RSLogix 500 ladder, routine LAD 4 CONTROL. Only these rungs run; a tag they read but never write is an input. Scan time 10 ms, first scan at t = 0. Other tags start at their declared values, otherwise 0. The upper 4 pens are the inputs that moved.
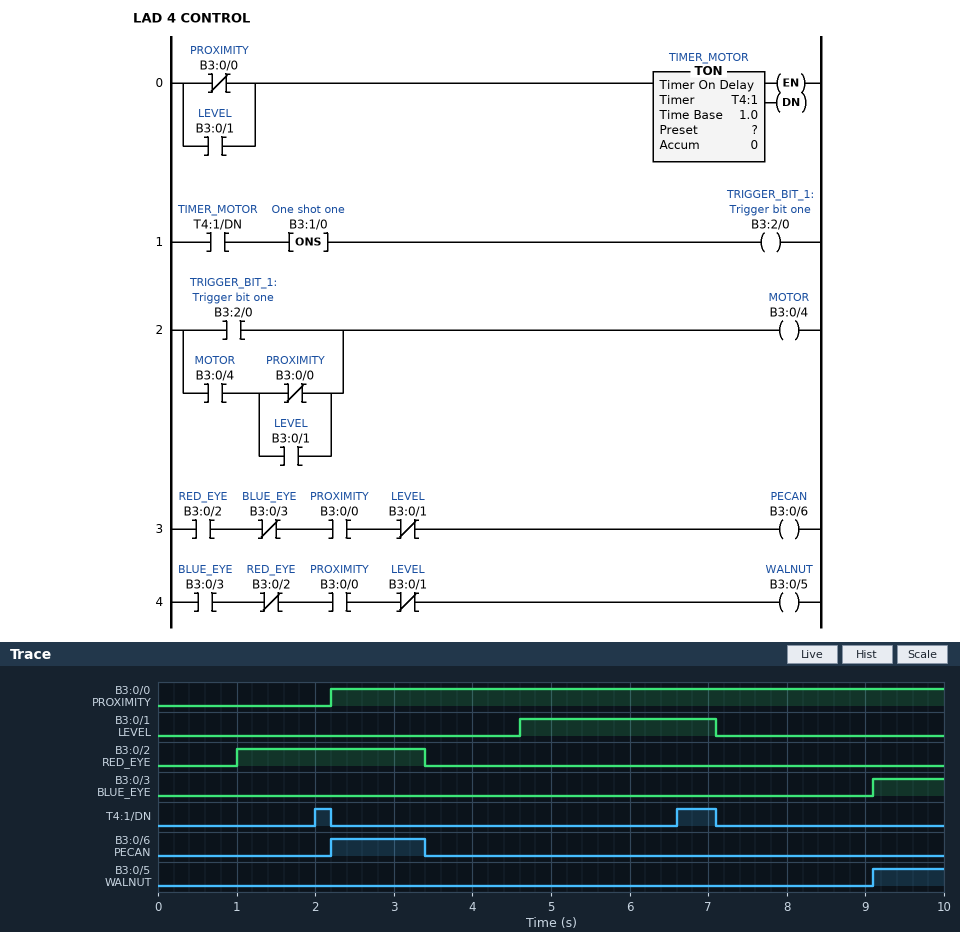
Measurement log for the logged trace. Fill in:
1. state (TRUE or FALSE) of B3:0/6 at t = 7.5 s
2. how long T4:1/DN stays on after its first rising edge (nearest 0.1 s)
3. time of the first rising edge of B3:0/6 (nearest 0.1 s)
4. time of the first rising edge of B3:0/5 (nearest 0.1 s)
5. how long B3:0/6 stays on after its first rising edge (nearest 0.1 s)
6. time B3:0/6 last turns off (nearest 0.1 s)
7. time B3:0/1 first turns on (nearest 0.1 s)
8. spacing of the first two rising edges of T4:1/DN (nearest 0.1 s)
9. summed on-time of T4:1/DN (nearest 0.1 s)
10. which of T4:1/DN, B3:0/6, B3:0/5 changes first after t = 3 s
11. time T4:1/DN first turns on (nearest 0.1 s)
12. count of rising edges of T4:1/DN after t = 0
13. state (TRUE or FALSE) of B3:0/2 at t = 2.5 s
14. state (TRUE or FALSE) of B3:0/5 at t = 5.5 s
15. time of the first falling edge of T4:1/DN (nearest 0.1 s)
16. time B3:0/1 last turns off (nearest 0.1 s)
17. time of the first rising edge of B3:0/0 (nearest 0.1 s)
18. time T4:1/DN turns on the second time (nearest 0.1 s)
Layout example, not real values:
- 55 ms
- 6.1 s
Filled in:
- FALSE
- 0.2 s
- 2.2 s
- 9.1 s
- 1.2 s
- 3.4 s
- 4.6 s
- 4.6 s
- 0.7 s
- B3:0/6
- 2.0 s
- 2
- TRUE
- FALSE
- 2.2 s
- 7.1 s
- 2.2 s
- 6.6 s
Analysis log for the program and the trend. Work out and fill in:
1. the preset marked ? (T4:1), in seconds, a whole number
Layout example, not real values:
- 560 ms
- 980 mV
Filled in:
- 2 s
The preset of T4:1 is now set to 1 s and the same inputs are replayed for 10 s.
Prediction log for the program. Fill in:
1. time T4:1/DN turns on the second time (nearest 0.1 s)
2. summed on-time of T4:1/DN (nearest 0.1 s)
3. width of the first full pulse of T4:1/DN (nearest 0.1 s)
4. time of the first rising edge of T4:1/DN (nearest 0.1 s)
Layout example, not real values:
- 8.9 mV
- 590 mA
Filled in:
- 5.6 s
- 2.7 s
- 1.2 s
- 1.0 s
